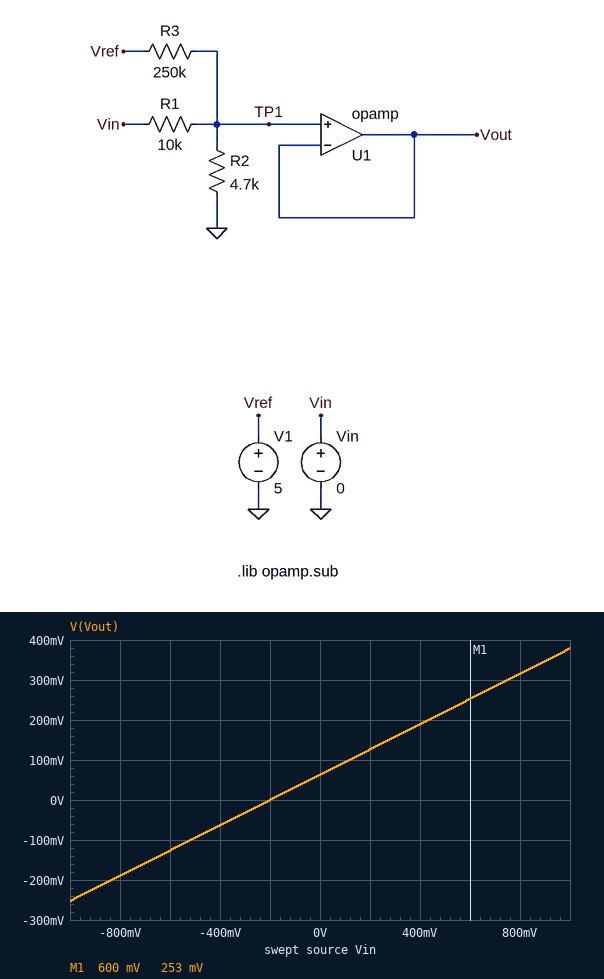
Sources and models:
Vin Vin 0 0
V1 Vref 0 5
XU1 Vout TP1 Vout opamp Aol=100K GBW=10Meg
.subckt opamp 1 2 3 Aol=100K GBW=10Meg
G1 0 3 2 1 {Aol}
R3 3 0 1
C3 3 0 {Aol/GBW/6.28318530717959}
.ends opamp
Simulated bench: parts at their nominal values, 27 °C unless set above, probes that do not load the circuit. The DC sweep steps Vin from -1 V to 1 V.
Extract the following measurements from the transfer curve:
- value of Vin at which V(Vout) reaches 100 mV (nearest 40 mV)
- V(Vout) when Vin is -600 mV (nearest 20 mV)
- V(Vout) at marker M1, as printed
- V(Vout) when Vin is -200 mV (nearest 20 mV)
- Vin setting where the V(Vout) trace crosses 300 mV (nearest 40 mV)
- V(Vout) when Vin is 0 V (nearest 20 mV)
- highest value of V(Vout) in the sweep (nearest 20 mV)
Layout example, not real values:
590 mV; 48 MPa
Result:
120 mV; -120 mV; 253 mV; 0 V; 760 mV; 60 mV; 380 mV
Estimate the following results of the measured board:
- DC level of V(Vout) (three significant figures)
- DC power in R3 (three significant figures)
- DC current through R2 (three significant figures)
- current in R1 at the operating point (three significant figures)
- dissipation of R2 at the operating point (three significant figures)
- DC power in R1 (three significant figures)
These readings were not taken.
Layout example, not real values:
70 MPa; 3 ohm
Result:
63.1 mV; 97.5 µW; 13.4 µA; 6.31 µA; 848 nW; 399 nW
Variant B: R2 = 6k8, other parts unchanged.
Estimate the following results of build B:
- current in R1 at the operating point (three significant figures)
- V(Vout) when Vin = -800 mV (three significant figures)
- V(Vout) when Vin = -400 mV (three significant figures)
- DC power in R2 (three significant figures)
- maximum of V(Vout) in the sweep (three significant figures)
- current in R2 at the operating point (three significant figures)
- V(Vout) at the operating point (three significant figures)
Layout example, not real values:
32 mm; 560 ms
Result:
7.97 µA; -239 mV; -79.7 mV; 933 nW; 478 mV; 11.7 µA; 79.7 mV
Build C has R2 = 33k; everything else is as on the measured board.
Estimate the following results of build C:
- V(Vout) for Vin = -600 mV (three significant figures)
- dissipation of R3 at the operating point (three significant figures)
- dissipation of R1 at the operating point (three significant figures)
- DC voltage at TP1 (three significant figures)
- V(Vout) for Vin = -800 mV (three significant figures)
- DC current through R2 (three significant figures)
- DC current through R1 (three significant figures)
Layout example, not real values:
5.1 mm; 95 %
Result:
-298 mV; 94.1 µW; 2.22 µW; 149 mV; -447 mV; 4.51 µA; 14.9 µA
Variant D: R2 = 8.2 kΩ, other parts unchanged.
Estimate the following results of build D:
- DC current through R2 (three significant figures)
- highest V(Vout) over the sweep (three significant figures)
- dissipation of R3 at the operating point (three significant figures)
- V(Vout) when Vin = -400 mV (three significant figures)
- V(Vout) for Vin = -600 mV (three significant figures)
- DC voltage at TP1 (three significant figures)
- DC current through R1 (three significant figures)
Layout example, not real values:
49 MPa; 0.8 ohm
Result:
10.8 µA; 531 mV; 96.5 µW; -88.5 mV; -177 mV; 88.5 mV; 8.85 µA
